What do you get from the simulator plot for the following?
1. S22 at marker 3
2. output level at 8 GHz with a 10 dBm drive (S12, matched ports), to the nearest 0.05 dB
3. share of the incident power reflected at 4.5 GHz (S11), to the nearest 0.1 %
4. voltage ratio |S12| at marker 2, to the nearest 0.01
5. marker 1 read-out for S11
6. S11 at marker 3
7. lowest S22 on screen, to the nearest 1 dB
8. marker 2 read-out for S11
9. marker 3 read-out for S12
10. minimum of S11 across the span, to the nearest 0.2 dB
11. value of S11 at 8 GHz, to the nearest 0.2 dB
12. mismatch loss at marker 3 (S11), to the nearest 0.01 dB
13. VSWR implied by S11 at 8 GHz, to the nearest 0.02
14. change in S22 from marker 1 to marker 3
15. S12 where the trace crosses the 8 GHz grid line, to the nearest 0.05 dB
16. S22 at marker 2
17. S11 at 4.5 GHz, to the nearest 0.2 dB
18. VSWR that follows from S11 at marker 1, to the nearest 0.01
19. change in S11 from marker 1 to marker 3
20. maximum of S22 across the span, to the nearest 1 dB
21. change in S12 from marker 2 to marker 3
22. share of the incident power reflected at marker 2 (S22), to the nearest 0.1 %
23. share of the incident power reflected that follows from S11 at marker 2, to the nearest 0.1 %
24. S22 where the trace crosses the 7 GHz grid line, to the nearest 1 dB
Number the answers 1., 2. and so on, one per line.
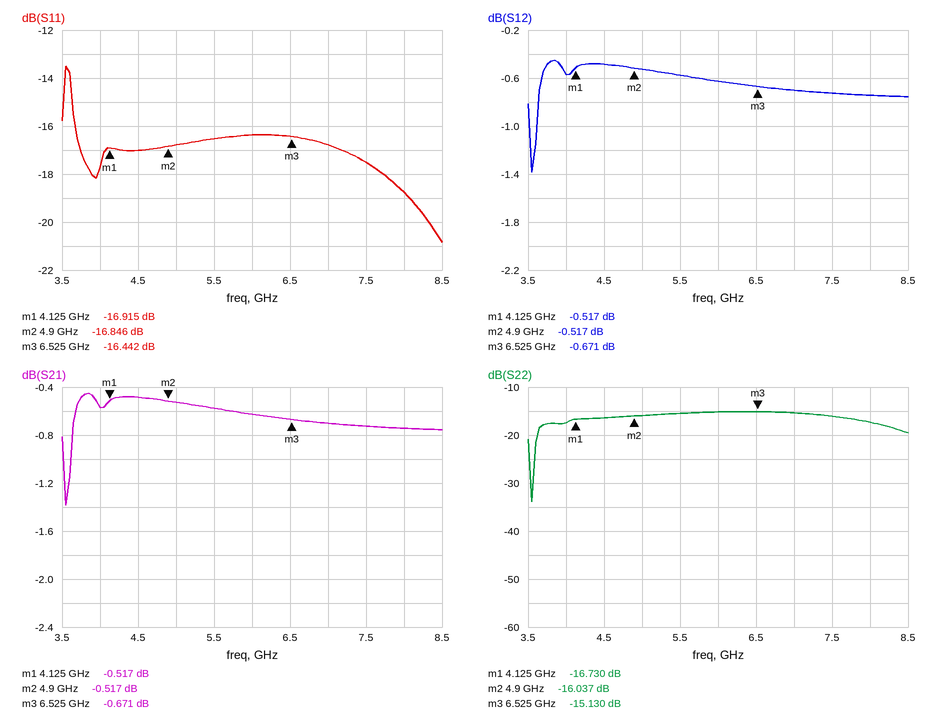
1. -15.130 dB
2. 9.25 dBm
3. 2.0 %
4. 0.94
5. -16.915 dB
6. -16.442 dB
7. -34 dB
8. -16.846 dB
9. -0.671 dB
10. -20.8 dB
11. -18.8 dB
12. 0.10 dB
13. 1.26
14. 1.600 dB
15. -0.75 dB
16. -16.037 dB
17. -17.0 dB
18. 1.33
19. 0.473 dB
20. -15 dB
21. -0.154 dB
22. 2.5 %
23. 2.1 %
24. -15 dB
